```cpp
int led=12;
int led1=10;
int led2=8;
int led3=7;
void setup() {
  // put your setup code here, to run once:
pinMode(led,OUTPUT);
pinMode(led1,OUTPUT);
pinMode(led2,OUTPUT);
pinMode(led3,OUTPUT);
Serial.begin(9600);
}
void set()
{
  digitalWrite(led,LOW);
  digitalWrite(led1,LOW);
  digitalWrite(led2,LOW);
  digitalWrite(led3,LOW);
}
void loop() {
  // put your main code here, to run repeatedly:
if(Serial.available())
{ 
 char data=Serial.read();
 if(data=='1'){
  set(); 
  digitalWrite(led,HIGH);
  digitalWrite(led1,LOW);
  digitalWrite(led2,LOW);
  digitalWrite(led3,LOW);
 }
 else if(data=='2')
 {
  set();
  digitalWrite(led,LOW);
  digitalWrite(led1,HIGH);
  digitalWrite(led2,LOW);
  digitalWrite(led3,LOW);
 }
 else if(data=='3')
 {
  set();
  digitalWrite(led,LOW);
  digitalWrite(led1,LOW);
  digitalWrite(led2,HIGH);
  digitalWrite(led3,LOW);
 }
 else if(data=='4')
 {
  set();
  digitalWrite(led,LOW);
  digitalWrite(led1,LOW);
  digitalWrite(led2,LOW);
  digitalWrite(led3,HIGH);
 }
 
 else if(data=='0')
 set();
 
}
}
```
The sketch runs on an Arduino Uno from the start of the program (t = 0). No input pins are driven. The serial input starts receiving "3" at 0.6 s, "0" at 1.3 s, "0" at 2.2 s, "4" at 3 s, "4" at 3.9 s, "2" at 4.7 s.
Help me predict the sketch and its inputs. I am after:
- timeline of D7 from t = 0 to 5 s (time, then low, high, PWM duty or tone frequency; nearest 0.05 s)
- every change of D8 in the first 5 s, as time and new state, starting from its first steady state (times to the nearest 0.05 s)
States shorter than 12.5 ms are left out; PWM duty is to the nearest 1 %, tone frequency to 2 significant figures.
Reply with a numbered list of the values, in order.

1. 0 s low; 3 s high; 4.7 s low
2. 0 s low; 0.6 s high; 1.3 s low
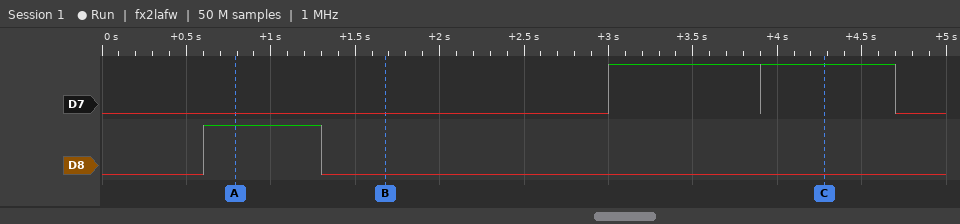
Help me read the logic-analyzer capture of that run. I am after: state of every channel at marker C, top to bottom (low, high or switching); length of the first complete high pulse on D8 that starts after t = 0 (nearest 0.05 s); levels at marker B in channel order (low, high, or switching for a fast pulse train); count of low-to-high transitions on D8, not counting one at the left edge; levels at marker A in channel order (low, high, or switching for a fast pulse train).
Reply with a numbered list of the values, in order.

1. D7 high, D8 low
2. 0.70 s
3. D7 low, D8 low
4. 1
5. D7 low, D8 high
